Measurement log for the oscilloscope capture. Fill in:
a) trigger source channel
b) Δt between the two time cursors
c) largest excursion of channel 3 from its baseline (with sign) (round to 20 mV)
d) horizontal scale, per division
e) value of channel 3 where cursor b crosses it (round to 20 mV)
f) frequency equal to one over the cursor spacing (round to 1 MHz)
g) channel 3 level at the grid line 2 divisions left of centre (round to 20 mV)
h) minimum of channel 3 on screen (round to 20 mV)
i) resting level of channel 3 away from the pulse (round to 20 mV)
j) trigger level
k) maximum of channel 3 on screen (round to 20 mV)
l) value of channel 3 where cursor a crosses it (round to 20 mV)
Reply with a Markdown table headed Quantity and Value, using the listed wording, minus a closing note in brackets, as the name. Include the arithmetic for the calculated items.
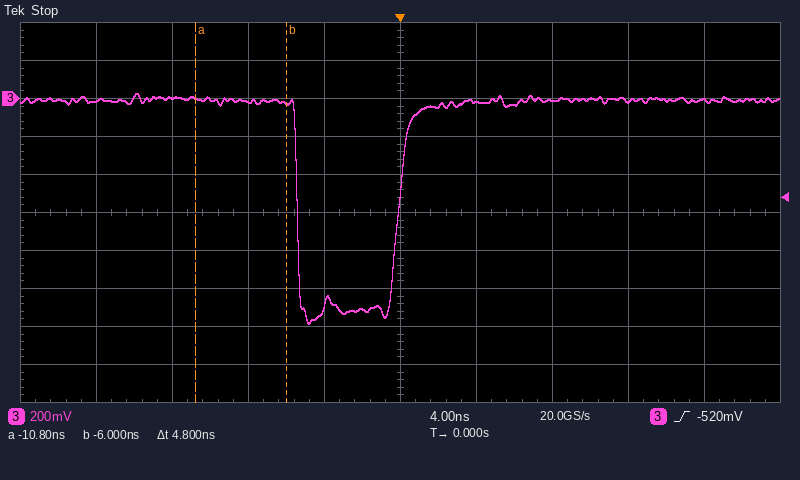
| Quantity | Value |
|---|---|
| trigger source channel | channel 3 |
| Δt between the two time cursors | 4.8 ns |
| largest excursion of channel 3 from its baseline (with sign) | -1.18 V − (0 mV) = -1.18 V |
| horizontal scale, per division | 4 ns |
| value of channel 3 where cursor b crosses it | -20 mV |
| frequency equal to one over the cursor spacing | 1 / 4.8 ns ≈ 208 MHz |
| channel 3 level at the grid line 2 divisions left of centre | -20 mV |
| minimum of channel 3 on screen | -1.18 V |
| resting level of channel 3 away from the pulse | 0 mV |
| trigger level | -520 mV |
| maximum of channel 3 on screen | 20 mV |
| value of channel 3 where cursor a crosses it | 0 mV |
